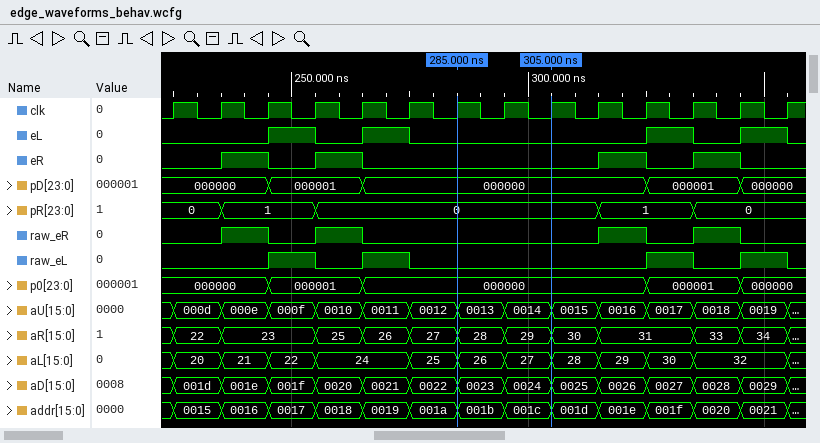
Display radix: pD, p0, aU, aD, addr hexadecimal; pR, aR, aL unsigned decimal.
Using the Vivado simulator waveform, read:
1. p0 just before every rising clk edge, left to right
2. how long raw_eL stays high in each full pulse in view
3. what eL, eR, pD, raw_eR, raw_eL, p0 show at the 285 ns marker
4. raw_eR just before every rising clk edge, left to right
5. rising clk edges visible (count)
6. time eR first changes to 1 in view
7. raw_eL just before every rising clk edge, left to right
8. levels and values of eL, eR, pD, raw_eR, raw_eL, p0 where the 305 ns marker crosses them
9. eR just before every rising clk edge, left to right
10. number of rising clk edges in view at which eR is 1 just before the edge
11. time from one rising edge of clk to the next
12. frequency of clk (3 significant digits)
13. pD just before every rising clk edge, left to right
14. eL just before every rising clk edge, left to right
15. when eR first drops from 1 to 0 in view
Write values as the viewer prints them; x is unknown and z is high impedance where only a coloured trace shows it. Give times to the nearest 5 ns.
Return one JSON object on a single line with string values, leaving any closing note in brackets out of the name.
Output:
{"p0 just before every rising clk edge, left to right": "000000, 000000, 000000, 000001, 000001, 000000, 000000, 000000, 000000, 000000, 000000, 000001, 000001, 000000", "how long raw_eL stays high in each full pulse in view": "10 ns, 10 ns, 10 ns, 10 ns", "what eL, eR, pD, raw_eR, raw_eL, p0 show at the 285 ns marker": "eL=0, eR=0, pD=000000, raw_eR=0, raw_eL=0, p0=000000", "raw_eR just before every rising clk edge, left to right": "0 0 1 0 1 0 0 0 0 0 1 0 1 0", "rising clk edges visible": "14", "time eR first changes to 1 in view": "235 ns", "raw_eL just before every rising clk edge, left to right": "0 0 0 1 0 1 0 0 0 0 0 1 0 1", "levels and values of eL, eR, pD, raw_eR, raw_eL, p0 where the 305 ns marker crosses them": "eL=0, eR=0, pD=000000, raw_eR=0, raw_eL=0, p0=000000", "eR just before every rising clk edge, left to right": "0 0 1 0 1 0 0 0 0 0 1 0 1 0", "number of rising clk edges in view at which eR is 1 just before the edge": "4", "time from one rising edge of clk to the next": "10 ns", "frequency of clk": "100 MHz", "pD just before every rising clk edge, left to right": "000000, 000000, 000000, 000001, 000001, 000000, 000000, 000000, 000000, 000000, 000000, 000001, 000001, 000000", "eL just before every rising clk edge, left to right": "0 0 0 1 0 1 0 0 0 0 0 1 0 1", "when eR first drops from 1 to 0 in view": "245 ns"}
